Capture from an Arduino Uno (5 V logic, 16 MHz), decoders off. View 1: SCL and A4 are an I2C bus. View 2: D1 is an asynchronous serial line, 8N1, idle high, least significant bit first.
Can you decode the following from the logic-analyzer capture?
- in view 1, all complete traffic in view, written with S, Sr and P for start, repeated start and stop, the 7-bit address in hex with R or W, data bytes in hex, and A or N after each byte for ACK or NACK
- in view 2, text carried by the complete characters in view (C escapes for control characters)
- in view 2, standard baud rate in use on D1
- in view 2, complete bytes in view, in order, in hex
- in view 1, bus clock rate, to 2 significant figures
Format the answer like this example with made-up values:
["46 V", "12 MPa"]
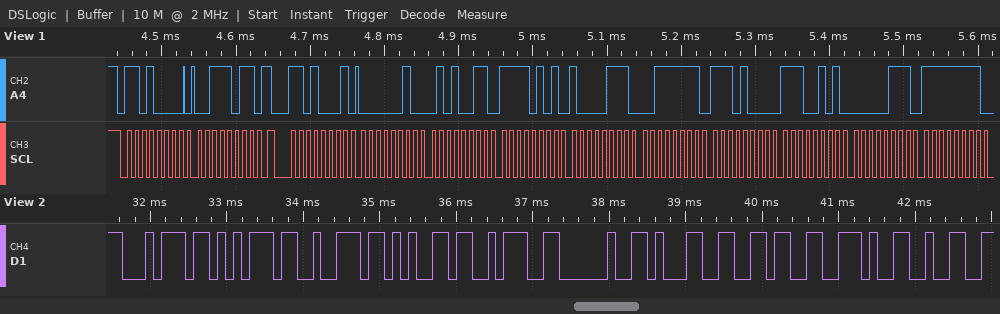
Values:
["S 68W A 3B A Sr 68R A 02 A 53 A F5 A 87 A 3F A E8 A E5 A 07 A FF A", "\"ture: 16.2\"", "9600 baud", "0x74 0x75 0x72 0x65 0x3A 0x20 0x31 0x36 0x2E 0x32", "100 kHz"]
